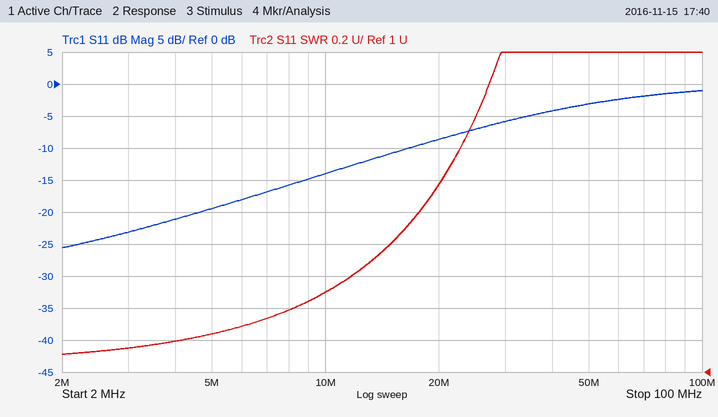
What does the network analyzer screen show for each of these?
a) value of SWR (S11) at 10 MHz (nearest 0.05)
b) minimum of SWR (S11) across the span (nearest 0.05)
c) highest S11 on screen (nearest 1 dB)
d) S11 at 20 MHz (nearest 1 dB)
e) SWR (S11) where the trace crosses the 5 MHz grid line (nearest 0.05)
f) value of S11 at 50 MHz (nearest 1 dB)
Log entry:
1.50
1.10
-1 dB
-9 dB
1.25
-3 dB
